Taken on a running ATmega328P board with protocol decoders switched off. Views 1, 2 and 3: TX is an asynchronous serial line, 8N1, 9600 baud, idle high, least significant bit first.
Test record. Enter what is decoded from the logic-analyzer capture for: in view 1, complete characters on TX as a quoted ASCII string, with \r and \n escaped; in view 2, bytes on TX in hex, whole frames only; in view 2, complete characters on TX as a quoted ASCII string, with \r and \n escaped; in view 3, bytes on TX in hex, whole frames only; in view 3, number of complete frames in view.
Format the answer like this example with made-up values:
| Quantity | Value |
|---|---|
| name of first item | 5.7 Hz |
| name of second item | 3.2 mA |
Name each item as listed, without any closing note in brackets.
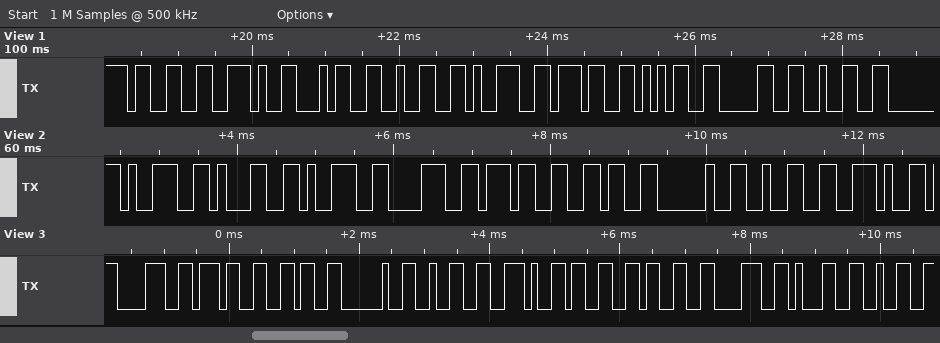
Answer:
| Quantity | Value |
|---|---|
| in view 1, complete characters on TX as a quoted ASCII string, with \r and \n escaped | "3.4297502" |
| in view 2, bytes on TX in hex, whole frames only | 0x39 0x31 0x39 0x38 0x37 0x36 0x20 0x32 0x2E |
| in view 2, complete characters on TX as a quoted ASCII string, with \r and \n escaped | "919876 2." |
| in view 3, bytes on TX in hex, whole frames only | 38 37 36 20 32 2E 33 33 38 31 32 |
| in view 3, number of complete frames in view | 11 |
